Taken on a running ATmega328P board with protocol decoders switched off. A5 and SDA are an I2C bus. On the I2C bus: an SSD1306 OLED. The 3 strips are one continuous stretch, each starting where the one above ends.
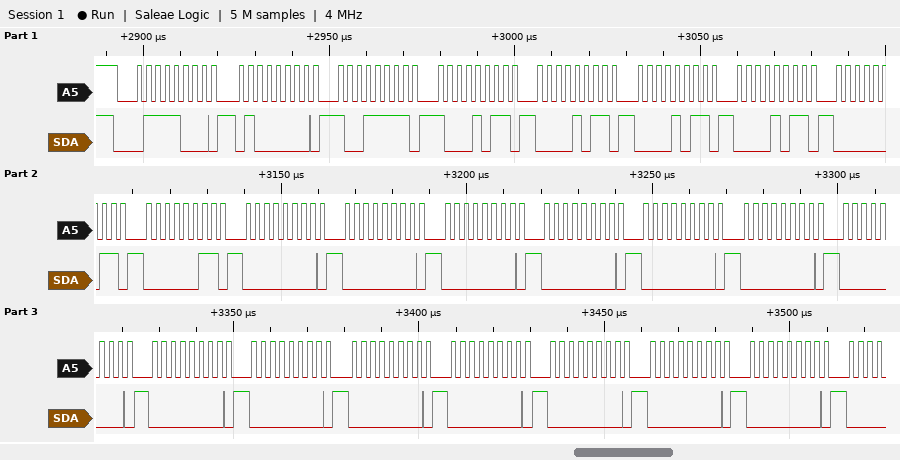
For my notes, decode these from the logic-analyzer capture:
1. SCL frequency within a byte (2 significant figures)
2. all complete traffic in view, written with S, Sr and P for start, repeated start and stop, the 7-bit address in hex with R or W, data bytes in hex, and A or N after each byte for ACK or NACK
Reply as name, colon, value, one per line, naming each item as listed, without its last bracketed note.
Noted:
SCL frequency within a byte: 400 kHz
all complete traffic in view, written with S, Sr and P for start, repeated start and stop, the 7-bit address in hex with R or W, data bytes in hex, and A or N after each byte for ACK or NACK: S 3CW A 40 A 9F A 8B A 0B A 0B A 0B A 03 A 03 A 00 A 00 A 00 A 00 A 00 A 00 A 00 A 00 A 00 A 00 A 00 A 00 A 00 A 00 A
